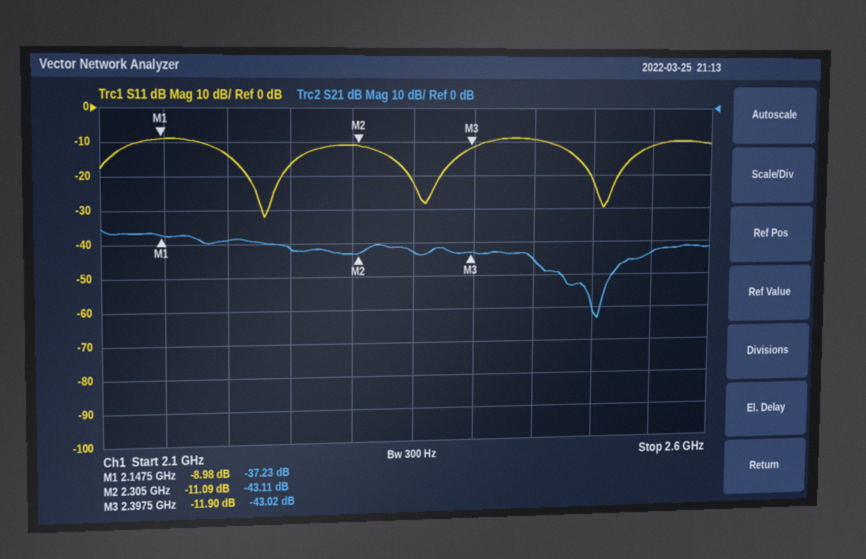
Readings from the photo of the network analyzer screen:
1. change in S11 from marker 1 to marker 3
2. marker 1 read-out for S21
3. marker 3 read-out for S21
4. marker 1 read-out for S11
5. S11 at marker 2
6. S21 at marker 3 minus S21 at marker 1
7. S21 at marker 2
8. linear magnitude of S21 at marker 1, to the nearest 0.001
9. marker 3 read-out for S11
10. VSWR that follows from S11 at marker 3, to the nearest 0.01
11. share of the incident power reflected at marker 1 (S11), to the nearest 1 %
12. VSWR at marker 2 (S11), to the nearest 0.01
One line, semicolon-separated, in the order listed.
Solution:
-2.92 dB; -37.23 dB; -43.02 dB; -8.98 dB; -11.09 dB; -5.79 dB; -43.11 dB; 0.014; -11.90 dB; 1.68; 13 %; 1.77
